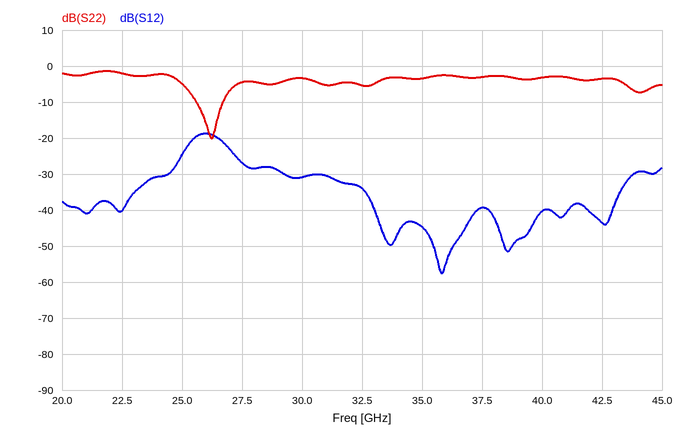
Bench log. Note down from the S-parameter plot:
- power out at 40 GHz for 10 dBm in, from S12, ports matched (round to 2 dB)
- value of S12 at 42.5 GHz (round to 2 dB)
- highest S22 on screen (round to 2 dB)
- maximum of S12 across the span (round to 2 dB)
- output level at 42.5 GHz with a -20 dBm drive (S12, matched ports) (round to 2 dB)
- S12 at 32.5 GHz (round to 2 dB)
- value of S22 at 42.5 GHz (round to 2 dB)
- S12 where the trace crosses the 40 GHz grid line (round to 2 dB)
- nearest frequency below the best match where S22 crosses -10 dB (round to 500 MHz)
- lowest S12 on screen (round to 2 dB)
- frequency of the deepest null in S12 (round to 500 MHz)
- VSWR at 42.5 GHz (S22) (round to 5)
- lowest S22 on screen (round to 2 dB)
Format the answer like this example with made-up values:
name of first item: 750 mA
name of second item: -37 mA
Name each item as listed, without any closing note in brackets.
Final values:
power out at 40 GHz for 10 dBm in, from S12, ports matched: -30 dBm
value of S12 at 42.5 GHz: -44 dB
highest S22 on screen: -2 dB
maximum of S12 across the span: -18 dB
output level at 42.5 GHz with a -20 dBm drive (S12, matched ports): -64 dBm
S12 at 32.5 GHz: -34 dB
value of S22 at 42.5 GHz: -4 dB
S12 where the trace crosses the 40 GHz grid line: -40 dB
nearest frequency below the best match where S22 crosses -10 dB: 25.5 GHz
lowest S12 on screen: -58 dB
frequency of the deepest null in S12: 36.0 GHz
VSWR at 42.5 GHz (S22): 5
lowest S22 on screen: -20 dB
